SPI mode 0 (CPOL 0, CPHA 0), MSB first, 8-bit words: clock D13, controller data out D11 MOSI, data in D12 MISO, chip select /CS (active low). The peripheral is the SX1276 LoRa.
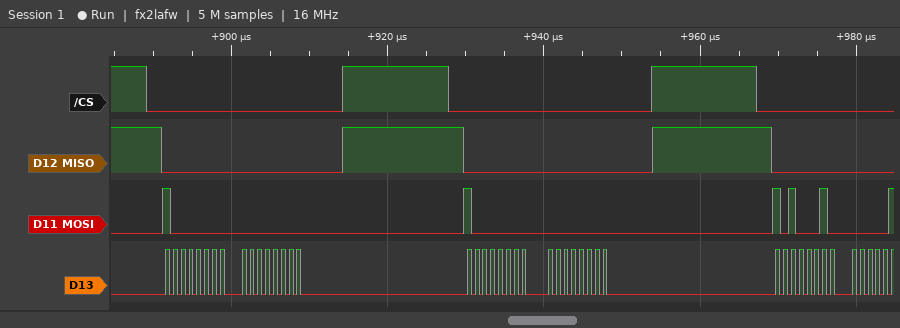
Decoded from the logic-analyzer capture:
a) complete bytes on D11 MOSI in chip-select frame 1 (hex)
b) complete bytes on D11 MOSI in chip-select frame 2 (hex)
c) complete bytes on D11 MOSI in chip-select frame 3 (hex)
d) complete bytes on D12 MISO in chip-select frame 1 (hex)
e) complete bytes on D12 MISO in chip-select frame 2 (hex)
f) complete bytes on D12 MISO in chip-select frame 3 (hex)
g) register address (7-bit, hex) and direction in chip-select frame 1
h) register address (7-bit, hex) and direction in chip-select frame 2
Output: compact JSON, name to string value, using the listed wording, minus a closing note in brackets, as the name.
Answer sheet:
{"complete bytes on D11 MOSI in chip-select frame 1": "80 00", "complete bytes on D11 MOSI in chip-select frame 2": "80 00", "complete bytes on D11 MOSI in chip-select frame 3": "A2", "complete bytes on D12 MISO in chip-select frame 1": "00 00", "complete bytes on D12 MISO in chip-select frame 2": "00 00", "complete bytes on D12 MISO in chip-select frame 3": "00", "register address (7-bit, hex) and direction in chip-select frame 1": "0x00 write", "register address (7-bit, hex) and direction in chip-select frame 2": "0x00 write"}
